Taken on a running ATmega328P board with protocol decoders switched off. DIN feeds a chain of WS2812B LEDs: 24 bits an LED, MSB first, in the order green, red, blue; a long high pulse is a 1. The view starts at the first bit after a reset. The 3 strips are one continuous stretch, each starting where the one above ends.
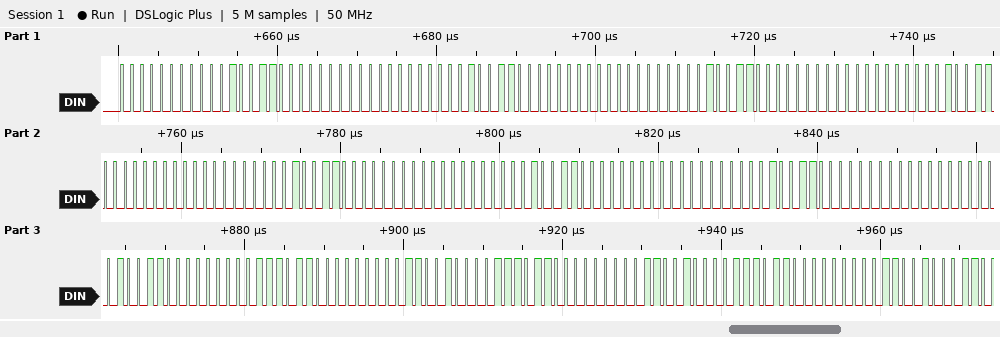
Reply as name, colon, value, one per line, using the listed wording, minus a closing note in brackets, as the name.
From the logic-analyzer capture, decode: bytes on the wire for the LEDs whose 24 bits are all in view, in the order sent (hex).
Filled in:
bytes on the wire for the LEDs whose 24 bits are all in view, in the order sent: 00 13 00 00 13 00 00 13 00 00 13 00 00 13 00 00 13 00 00 13 00 00 13 00 76 00 C8 76 00 C8 76 00 C8
